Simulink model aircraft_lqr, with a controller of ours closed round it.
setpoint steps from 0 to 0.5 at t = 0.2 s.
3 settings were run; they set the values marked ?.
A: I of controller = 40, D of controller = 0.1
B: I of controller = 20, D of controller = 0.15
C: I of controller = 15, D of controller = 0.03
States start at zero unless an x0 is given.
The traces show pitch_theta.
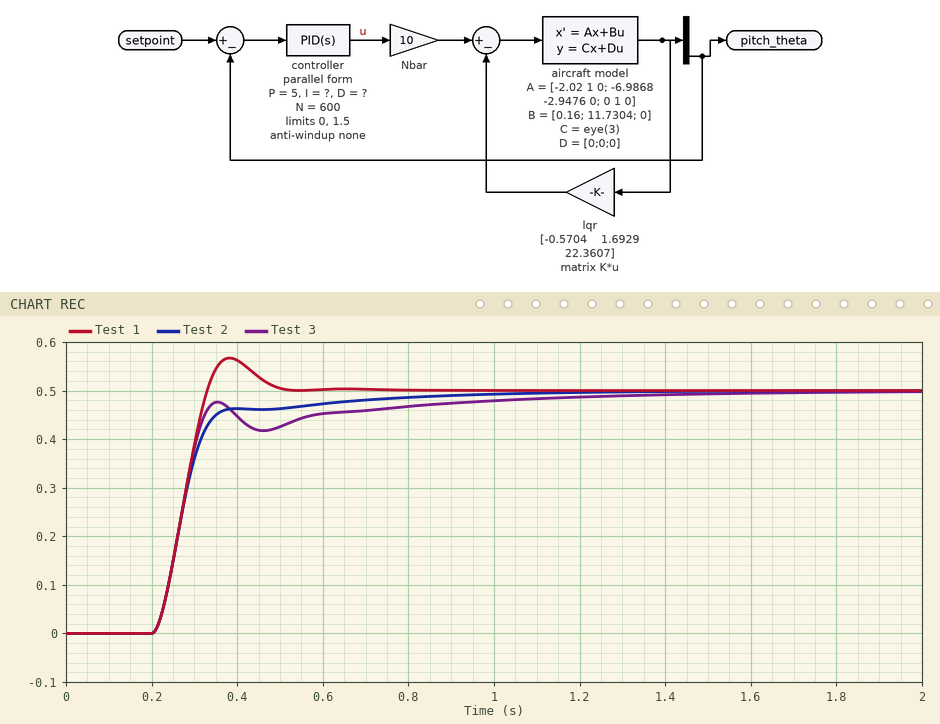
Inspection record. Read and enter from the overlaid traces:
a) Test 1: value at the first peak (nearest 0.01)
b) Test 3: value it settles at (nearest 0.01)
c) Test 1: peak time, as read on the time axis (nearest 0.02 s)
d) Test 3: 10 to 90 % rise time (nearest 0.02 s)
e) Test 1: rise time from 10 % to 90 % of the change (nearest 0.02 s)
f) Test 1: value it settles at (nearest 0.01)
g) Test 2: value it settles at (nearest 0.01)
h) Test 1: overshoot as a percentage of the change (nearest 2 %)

0.57
0.50
0.38 s
0.10 s
0.08 s
0.50
0.50
14 %
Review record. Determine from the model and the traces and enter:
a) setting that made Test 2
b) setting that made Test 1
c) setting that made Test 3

B
A
C
